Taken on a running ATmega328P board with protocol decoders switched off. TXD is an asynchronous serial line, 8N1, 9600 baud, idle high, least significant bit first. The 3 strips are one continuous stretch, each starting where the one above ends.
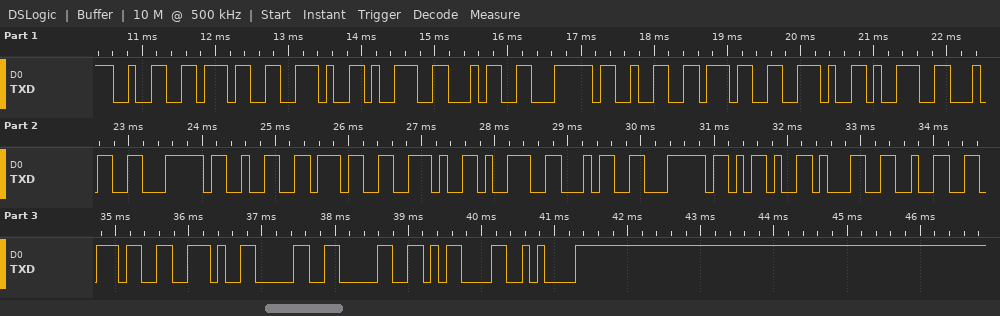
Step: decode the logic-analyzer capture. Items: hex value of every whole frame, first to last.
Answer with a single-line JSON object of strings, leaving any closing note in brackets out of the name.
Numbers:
{"hex value of every whole frame, first to last": "32 37 2E 39 34 7C 32 37 2E 39 34 7C 32 37 2E 39 34 7C 2D 31 32 37 2E 30 30 0D 0A"}
